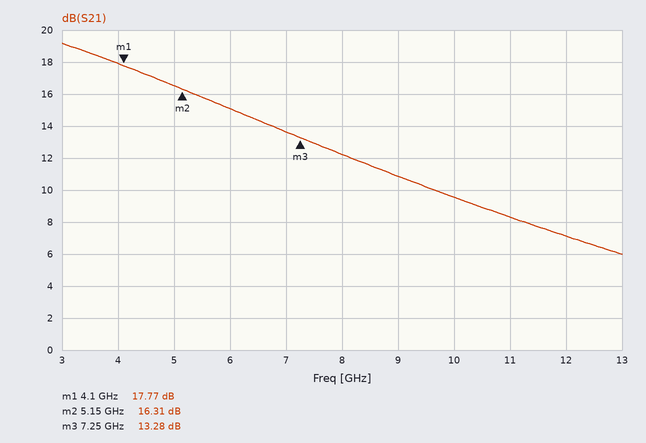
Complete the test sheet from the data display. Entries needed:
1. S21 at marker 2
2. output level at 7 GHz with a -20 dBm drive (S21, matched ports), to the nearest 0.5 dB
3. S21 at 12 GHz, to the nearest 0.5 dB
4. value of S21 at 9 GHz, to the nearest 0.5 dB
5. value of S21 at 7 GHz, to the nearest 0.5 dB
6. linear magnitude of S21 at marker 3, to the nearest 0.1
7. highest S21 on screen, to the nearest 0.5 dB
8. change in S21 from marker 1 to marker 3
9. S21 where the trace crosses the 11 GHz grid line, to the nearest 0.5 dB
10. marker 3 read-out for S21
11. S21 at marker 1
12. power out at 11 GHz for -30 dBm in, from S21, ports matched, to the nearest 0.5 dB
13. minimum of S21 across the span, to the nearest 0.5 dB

16.31 dB
-6.5 dBm
7.0 dB
11.0 dB
13.5 dB
4.6
19.0 dB
-4.49 dB
8.5 dB
13.28 dB
17.77 dB
-21.5 dBm
6.0 dB
